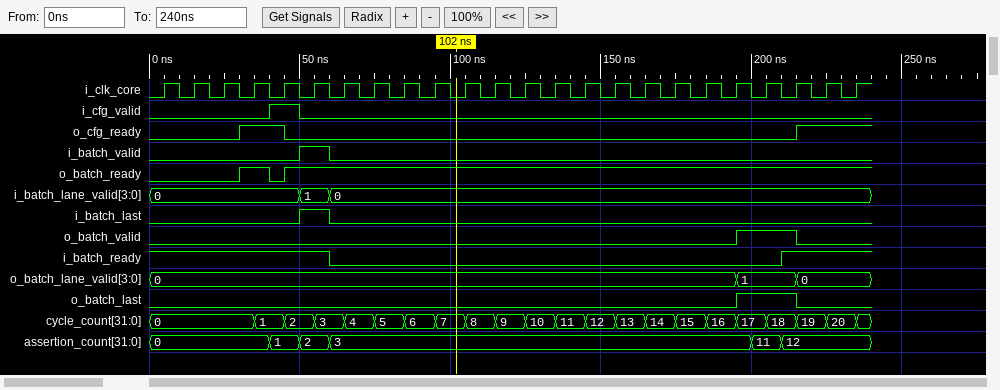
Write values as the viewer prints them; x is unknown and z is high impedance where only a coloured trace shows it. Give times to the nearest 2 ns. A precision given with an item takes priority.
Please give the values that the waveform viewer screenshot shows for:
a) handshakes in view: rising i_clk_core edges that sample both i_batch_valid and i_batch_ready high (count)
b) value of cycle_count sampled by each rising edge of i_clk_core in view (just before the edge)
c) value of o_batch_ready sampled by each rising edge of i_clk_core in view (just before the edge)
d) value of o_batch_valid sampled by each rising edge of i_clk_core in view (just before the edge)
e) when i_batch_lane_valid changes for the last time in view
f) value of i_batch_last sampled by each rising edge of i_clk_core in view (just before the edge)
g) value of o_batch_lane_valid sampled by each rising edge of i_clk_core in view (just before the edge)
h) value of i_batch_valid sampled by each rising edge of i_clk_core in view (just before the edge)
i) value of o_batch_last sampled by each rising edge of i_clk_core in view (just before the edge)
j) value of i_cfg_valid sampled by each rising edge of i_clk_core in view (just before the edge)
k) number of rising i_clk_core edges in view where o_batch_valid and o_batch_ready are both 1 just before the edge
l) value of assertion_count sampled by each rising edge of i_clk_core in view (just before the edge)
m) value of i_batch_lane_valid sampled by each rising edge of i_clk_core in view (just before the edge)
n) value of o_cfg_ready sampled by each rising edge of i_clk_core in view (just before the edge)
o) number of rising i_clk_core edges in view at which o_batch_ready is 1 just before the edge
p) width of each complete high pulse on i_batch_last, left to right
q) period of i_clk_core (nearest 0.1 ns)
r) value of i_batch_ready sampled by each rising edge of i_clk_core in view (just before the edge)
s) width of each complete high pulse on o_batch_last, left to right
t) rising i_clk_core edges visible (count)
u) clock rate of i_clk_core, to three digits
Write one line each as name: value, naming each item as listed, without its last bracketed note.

handshakes in view: rising i_clk_core edges that sample both i_batch_valid and i_batch_ready high: 1
value of cycle_count sampled by each rising edge of i_clk_core in view: 0, 0, 0, 0, 1, 2, 3, 4, 5, 6, 7, 8, 9, 10, 11, 12, 13, 14, 15, 16, 17, 18, 19, 20
value of o_batch_ready sampled by each rising edge of i_clk_core in view: 0 0 0 1 0 1 1 1 1 1 1 1 1 1 1 1 1 1 1 1 1 1 1 1
value of o_batch_valid sampled by each rising edge of i_clk_core in view: 0 0 0 0 0 0 0 0 0 0 0 0 0 0 0 0 0 0 0 0 1 1 0 0
when i_batch_lane_valid changes for the last time in view: 60 ns
value of i_batch_last sampled by each rising edge of i_clk_core in view: 0 0 0 0 0 1 0 0 0 0 0 0 0 0 0 0 0 0 0 0 0 0 0 0
value of o_batch_lane_valid sampled by each rising edge of i_clk_core in view: 0, 0, 0, 0, 0, 0, 0, 0, 0, 0, 0, 0, 0, 0, 0, 0, 0, 0, 0, 0, 1, 1, 0, 0
value of i_batch_valid sampled by each rising edge of i_clk_core in view: 0 0 0 0 0 1 0 0 0 0 0 0 0 0 0 0 0 0 0 0 0 0 0 0
value of o_batch_last sampled by each rising edge of i_clk_core in view: 0 0 0 0 0 0 0 0 0 0 0 0 0 0 0 0 0 0 0 0 1 1 0 0
value of i_cfg_valid sampled by each rising edge of i_clk_core in view: 0 0 0 0 1 0 0 0 0 0 0 0 0 0 0 0 0 0 0 0 0 0 0 0
number of rising i_clk_core edges in view where o_batch_valid and o_batch_ready are both 1 just before the edge: 2
value of assertion_count sampled by each rising edge of i_clk_core in view: 0, 0, 0, 0, 1, 2, 3, 3, 3, 3, 3, 3, 3, 3, 3, 3, 3, 3, 3, 3, 11, 12, 12, 12
value of i_batch_lane_valid sampled by each rising edge of i_clk_core in view: 0, 0, 0, 0, 0, 1, 0, 0, 0, 0, 0, 0, 0, 0, 0, 0, 0, 0, 0, 0, 0, 0, 0, 0
value of o_cfg_ready sampled by each rising edge of i_clk_core in view: 0 0 0 1 1 0 0 0 0 0 0 0 0 0 0 0 0 0 0 0 0 0 1 1
number of rising i_clk_core edges in view at which o_batch_ready is 1 just before the edge: 20
width of each complete high pulse on i_batch_last, left to right: 10 ns
period of i_clk_core: 10 ns
value of i_batch_ready sampled by each rising edge of i_clk_core in view: 1 1 1 1 1 1 0 0 0 0 0 0 0 0 0 0 0 0 0 0 0 1 1 1
width of each complete high pulse on o_batch_last, left to right: 20 ns
rising i_clk_core edges visible: 24
clock rate of i_clk_core, to three digits: 100 MHz
